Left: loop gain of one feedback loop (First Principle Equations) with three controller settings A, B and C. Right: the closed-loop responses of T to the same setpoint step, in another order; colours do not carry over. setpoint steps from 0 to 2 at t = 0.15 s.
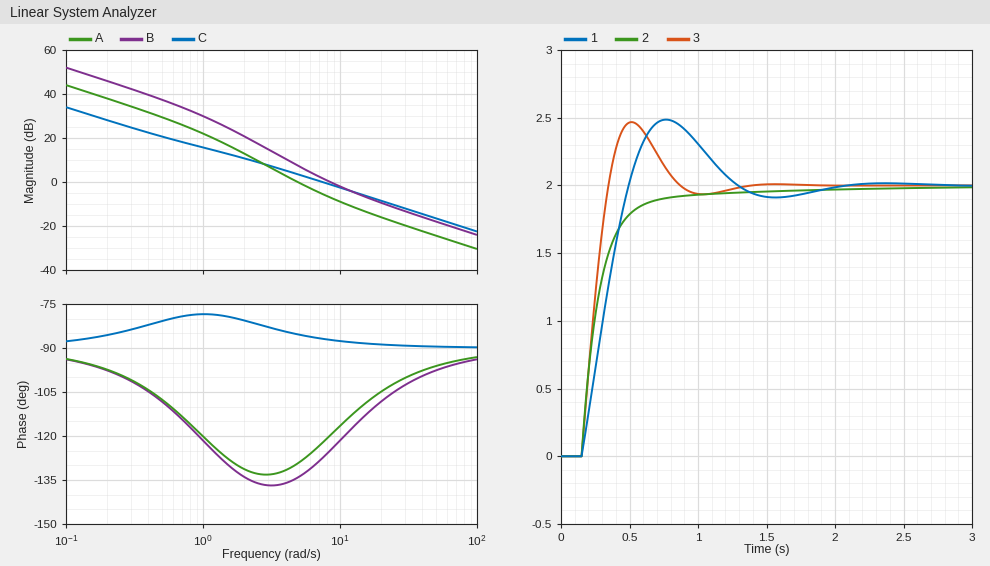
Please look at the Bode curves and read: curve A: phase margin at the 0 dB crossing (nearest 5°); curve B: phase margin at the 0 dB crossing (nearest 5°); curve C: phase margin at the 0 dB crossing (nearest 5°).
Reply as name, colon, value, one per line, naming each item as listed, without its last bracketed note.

curve A: phase margin at the 0 dB crossing: 50°
curve B: phase margin at the 0 dB crossing: 55°
curve C: phase margin at the 0 dB crossing: 95°
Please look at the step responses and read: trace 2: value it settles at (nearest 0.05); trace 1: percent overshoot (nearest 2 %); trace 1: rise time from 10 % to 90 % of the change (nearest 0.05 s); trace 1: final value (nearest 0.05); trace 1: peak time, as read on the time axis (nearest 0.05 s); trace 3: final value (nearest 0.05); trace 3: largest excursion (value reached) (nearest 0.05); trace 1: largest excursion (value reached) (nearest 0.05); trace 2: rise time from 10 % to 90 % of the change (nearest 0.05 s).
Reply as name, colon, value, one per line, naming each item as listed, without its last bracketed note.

trace 2: value it settles at: 2.00
trace 1: percent overshoot: 24 %
trace 1: rise time from 10 % to 90 % of the change: 0.25 s
trace 1: final value: 2.00
trace 1: peak time, as read on the time axis: 0.75 s
trace 3: final value: 2.00
trace 3: largest excursion (value reached): 2.45
trace 1: largest excursion (value reached): 2.50
trace 2: rise time from 10 % to 90 % of the change: 0.35 s
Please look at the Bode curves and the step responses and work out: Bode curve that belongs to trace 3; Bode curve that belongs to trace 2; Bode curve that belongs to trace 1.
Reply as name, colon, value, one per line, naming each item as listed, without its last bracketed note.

Bode curve that belongs to trace 3: B
Bode curve that belongs to trace 2: C
Bode curve that belongs to trace 1: A
